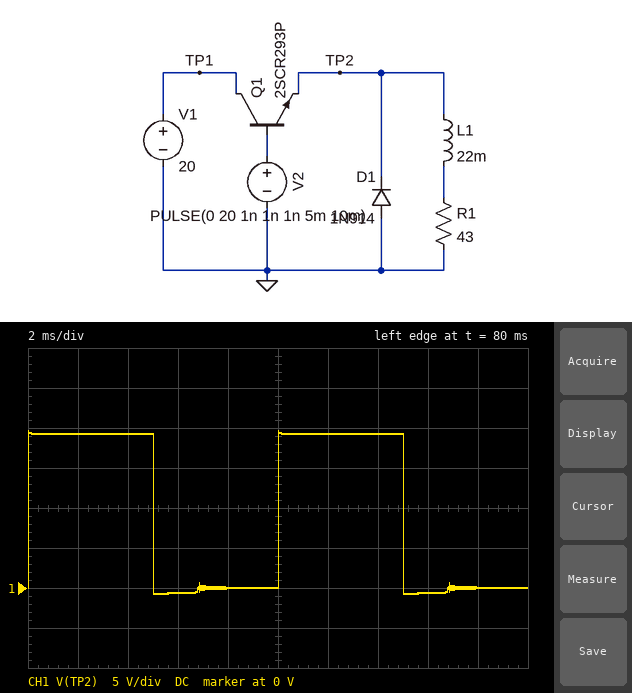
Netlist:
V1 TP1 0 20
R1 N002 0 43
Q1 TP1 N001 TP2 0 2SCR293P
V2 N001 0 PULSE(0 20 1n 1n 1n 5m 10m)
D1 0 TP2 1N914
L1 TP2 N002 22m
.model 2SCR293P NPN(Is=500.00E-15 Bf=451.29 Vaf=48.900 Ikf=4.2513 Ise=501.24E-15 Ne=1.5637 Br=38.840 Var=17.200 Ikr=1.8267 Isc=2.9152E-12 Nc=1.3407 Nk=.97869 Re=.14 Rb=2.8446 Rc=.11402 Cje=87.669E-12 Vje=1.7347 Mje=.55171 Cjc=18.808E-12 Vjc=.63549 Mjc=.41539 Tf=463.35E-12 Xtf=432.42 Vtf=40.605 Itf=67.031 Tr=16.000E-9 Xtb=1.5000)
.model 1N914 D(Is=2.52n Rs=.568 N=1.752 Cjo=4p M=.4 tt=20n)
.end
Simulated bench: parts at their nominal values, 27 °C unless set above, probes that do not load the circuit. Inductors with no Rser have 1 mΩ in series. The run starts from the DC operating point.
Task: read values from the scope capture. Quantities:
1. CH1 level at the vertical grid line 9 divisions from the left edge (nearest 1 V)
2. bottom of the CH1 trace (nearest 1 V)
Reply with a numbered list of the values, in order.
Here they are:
1. 0 V
2. -1 V
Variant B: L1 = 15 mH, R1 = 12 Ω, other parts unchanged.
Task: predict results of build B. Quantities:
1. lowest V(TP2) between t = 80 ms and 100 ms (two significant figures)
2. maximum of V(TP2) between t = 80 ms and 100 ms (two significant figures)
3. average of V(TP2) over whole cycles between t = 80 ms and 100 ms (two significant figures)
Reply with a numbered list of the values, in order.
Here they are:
1. -950 mV
2. 20 V
3. 9.2 V
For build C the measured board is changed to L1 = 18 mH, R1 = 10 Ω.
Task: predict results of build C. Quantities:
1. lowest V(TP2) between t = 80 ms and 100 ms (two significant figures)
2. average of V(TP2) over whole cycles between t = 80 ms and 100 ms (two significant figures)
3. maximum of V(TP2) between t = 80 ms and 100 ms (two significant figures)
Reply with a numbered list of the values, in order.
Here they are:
1. -980 mV
2. 9.1 V
3. 19 V
